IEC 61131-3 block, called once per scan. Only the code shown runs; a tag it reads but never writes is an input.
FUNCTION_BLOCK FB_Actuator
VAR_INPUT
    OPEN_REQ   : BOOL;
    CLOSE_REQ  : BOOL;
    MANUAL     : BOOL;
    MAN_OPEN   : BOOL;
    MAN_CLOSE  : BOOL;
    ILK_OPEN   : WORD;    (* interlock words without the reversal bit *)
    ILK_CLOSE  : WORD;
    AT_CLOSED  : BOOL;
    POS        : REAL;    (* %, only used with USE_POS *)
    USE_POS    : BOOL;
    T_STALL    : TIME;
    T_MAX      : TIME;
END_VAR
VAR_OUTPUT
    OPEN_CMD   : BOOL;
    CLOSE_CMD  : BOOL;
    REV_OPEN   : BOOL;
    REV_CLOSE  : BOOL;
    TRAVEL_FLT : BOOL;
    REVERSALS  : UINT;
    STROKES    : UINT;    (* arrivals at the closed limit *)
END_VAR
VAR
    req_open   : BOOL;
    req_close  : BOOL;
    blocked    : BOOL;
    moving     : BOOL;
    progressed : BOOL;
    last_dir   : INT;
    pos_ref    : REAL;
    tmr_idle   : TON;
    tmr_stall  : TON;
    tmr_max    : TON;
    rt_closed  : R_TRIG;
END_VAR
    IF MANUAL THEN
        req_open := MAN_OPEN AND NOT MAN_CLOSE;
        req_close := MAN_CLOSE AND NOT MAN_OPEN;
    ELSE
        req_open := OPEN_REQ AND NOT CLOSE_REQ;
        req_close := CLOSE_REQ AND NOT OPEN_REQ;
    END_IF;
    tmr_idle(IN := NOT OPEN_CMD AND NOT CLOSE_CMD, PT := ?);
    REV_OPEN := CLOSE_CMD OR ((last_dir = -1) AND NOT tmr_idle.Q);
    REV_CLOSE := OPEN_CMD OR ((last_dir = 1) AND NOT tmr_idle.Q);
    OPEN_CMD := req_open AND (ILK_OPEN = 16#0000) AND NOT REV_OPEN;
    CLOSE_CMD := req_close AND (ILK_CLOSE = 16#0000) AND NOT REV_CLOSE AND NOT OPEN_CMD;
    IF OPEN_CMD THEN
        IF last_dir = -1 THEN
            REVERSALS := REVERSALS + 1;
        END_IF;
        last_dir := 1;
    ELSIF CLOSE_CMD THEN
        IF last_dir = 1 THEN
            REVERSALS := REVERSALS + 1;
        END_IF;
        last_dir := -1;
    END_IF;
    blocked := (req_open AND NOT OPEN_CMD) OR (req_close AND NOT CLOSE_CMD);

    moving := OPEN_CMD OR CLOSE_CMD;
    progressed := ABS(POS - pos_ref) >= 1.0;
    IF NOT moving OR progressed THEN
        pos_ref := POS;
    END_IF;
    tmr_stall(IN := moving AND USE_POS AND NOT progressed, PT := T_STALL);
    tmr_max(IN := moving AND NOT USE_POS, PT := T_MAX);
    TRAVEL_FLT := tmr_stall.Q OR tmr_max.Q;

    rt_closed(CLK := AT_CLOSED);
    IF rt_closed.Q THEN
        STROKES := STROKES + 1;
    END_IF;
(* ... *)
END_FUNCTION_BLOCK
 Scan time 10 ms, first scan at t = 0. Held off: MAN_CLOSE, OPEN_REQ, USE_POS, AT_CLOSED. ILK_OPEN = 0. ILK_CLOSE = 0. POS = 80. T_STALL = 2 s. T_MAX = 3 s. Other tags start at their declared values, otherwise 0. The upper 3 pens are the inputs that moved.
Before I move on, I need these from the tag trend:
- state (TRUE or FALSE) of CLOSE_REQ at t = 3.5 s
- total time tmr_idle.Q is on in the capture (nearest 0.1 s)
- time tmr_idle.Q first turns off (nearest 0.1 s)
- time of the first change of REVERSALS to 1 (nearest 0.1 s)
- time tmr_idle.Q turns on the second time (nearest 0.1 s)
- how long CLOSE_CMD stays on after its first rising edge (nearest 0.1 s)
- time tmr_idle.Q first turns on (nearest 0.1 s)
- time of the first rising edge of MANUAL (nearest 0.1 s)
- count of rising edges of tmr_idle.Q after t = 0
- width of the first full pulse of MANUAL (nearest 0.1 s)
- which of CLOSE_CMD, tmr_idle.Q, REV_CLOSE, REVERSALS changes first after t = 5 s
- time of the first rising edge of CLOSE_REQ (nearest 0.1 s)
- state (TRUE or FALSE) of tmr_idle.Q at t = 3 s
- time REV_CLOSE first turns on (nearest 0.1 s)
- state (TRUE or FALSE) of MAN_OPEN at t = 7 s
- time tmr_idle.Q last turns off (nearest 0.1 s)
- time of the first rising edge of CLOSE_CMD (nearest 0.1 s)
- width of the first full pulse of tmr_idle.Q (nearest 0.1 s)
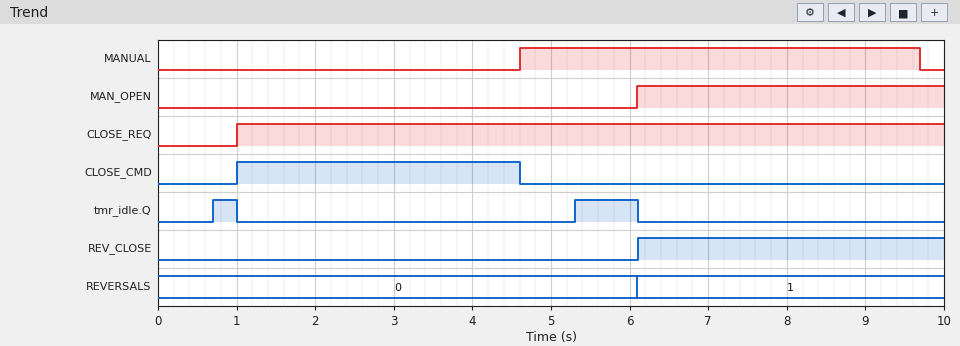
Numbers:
TRUE
1.1 s
1.0 s
6.1 s
5.3 s
3.6 s
0.7 s
4.6 s
2
5.1 s
tmr_idle.Q
1.0 s
FALSE
6.1 s
TRUE
6.1 s
1.0 s
0.3 s
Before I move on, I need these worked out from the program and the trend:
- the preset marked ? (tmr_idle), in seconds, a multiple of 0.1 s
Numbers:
0.7 s
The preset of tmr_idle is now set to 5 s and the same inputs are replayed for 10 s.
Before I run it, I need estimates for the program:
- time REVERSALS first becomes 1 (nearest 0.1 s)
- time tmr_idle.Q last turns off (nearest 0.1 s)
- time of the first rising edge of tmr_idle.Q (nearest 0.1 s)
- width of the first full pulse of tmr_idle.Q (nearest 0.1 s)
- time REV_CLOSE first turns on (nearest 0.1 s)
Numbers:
9.6 s
9.6 s
9.6 s
0.0 s
9.6 s
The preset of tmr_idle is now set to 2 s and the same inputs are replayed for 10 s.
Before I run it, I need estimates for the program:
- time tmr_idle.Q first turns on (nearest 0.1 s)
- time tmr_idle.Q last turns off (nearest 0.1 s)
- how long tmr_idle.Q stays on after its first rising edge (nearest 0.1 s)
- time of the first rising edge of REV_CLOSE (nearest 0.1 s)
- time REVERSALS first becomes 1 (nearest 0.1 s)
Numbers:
6.6 s
6.6 s
0.0 s
6.6 s
6.6 s
